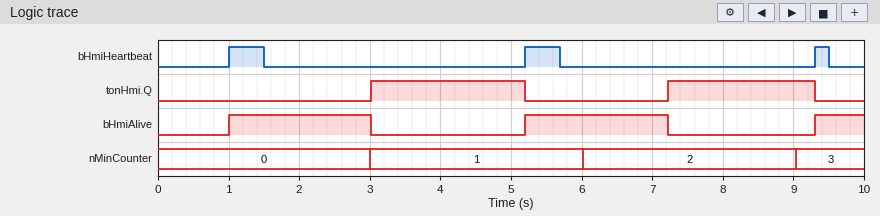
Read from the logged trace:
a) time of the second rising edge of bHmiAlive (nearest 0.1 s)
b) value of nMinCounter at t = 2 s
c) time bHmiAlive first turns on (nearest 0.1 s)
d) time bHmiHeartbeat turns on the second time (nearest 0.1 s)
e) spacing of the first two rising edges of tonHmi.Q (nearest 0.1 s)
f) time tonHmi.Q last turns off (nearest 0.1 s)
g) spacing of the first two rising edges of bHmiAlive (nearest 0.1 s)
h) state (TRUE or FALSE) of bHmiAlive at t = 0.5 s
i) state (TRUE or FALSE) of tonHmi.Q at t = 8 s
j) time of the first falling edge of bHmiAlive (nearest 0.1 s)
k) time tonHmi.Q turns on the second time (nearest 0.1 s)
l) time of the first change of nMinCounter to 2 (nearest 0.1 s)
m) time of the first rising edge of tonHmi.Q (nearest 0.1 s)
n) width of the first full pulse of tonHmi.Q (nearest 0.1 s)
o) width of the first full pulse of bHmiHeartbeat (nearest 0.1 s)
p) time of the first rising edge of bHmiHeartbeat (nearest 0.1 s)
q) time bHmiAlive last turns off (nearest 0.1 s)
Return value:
5.2 s
0
1.0 s
5.2 s
4.2 s
9.3 s
4.2 s
FALSE
TRUE
3.0 s
7.2 s
6.0 s
3.0 s
2.2 s
0.5 s
1.0 s
7.2 s
